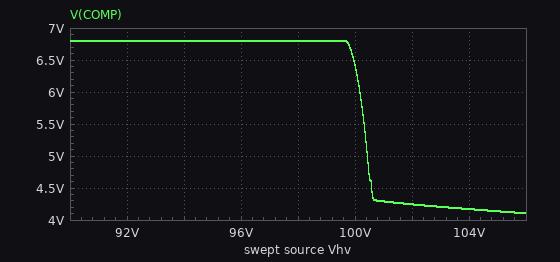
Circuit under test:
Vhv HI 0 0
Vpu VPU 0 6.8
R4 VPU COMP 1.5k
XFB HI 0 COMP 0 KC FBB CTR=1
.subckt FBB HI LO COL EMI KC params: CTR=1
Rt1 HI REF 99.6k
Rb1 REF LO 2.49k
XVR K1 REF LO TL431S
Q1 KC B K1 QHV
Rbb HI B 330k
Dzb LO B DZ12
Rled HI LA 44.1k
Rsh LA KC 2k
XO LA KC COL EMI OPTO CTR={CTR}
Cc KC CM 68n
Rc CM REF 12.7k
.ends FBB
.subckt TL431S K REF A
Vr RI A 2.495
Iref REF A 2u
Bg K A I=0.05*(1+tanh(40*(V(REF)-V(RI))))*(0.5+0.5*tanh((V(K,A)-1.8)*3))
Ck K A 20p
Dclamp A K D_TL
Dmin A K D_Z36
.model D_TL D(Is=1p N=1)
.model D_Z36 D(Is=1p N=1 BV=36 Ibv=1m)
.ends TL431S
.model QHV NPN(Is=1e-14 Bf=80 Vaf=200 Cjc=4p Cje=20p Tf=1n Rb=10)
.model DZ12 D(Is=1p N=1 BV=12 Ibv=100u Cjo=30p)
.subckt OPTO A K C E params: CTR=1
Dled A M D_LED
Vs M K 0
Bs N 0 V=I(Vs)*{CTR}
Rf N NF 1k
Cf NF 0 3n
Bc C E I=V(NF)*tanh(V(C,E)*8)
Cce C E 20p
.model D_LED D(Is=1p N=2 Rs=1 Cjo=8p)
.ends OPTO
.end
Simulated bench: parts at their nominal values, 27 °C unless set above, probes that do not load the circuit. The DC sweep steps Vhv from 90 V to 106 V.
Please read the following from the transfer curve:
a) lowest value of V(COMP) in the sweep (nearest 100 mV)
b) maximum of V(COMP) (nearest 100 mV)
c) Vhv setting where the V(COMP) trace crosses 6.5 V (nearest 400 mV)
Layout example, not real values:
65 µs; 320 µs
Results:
4.1 V; 6.8 V; 100.0 V
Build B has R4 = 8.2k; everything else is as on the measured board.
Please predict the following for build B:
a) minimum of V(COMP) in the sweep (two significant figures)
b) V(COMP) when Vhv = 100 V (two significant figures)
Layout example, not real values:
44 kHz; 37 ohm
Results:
62 mV; 4.7 V
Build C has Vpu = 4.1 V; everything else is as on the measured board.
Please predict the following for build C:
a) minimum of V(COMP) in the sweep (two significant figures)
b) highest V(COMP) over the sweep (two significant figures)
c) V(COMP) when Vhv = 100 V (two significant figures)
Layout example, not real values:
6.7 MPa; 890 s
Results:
1.4 V; 4.1 V; 3.7 V
